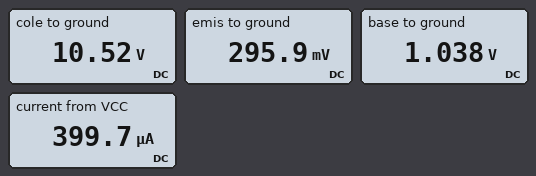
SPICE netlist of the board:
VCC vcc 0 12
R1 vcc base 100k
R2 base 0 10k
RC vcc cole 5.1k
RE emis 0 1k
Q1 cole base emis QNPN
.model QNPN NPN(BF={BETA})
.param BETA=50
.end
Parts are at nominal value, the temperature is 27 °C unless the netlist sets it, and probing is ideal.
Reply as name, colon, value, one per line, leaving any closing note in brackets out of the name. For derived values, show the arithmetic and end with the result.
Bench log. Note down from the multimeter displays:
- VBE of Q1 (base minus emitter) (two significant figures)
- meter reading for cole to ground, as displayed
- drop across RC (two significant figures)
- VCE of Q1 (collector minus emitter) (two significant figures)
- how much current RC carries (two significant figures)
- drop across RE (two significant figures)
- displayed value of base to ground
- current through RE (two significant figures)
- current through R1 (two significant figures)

VBE of Q1 (base minus emitter): 1.038 V - 295.9 mV = 740 mV
meter reading for cole to ground, as displayed: 10.52 V
drop across RC: 12 V - 10.52 V = 1.5 V
VCE of Q1 (collector minus emitter): 10.52 V - 295.9 mV = 10 V
how much current RC carries: (12 V - 10.52 V) / 5.1 kΩ = 290 µA
drop across RE: 295.9 mV = 300 mV
displayed value of base to ground: 1.038 V
current through RE: (295.9 mV) / 1 kΩ = 300 µA
current through R1: (12 V - 1.038 V) / 100 kΩ = 110 µA
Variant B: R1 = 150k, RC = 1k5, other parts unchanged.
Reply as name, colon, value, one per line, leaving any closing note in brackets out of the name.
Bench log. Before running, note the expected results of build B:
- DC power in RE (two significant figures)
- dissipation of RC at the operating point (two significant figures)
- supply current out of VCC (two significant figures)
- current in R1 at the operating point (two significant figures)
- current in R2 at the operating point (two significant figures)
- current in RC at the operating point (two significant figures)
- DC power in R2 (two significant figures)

DC power in RE: 2.2 µW
dissipation of RC at the operating point: 3.2 µW
supply current out of VCC: 120 µA
current in R1 at the operating point: 75 µA
current in R2 at the operating point: 74 µA
current in RC at the operating point: 46 µA
DC power in R2: 55 µW
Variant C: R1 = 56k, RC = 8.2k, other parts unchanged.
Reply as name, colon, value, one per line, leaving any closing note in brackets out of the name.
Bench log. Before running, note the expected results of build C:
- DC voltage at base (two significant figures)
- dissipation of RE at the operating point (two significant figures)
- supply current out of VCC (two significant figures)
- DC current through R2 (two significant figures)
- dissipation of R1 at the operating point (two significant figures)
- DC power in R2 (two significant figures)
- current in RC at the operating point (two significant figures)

DC voltage at base: 1.7 V
dissipation of RE at the operating point: 810 µW
supply current out of VCC: 1.1 mA
DC current through R2: 170 µA
dissipation of R1 at the operating point: 1.9 mW
DC power in R2: 280 µW
current in RC at the operating point: 880 µA
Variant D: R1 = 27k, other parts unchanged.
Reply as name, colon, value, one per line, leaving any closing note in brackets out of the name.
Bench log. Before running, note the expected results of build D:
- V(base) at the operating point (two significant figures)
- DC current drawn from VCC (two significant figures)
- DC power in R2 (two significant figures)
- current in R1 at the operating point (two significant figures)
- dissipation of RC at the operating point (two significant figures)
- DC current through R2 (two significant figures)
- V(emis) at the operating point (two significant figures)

V(base) at the operating point: 2.8 V
DC current drawn from VCC: 2.3 mA
DC power in R2: 780 µW
current in R1 at the operating point: 340 µA
dissipation of RC at the operating point: 19 mW
DC current through R2: 280 µA
V(emis) at the operating point: 2.0 V
